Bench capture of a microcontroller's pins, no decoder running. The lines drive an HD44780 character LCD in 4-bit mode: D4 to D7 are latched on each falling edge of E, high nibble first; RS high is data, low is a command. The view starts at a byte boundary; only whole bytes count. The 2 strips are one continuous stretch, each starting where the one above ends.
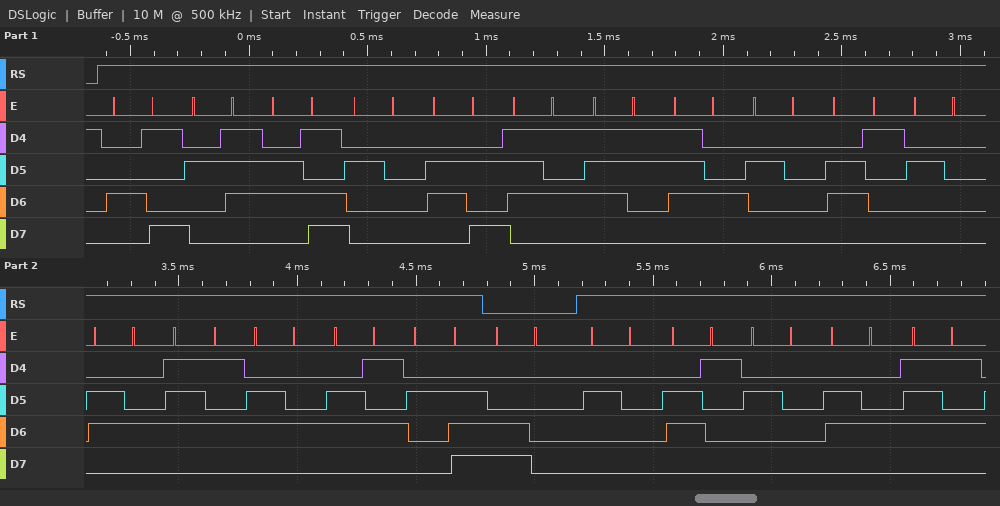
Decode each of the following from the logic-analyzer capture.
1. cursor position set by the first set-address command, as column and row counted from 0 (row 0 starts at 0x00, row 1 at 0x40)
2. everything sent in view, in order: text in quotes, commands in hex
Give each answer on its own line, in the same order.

column 0, row 1
"I'm just a dude." 0xC0 " a du"
